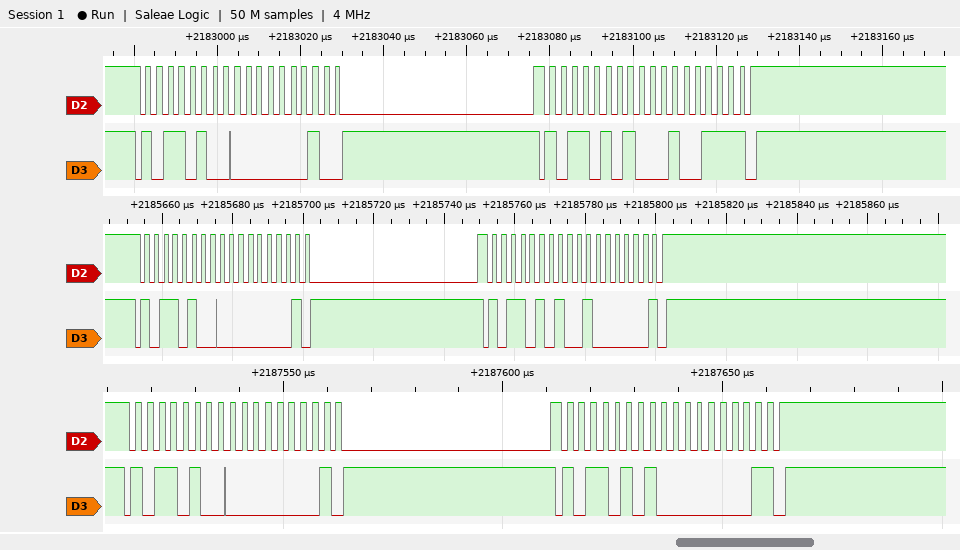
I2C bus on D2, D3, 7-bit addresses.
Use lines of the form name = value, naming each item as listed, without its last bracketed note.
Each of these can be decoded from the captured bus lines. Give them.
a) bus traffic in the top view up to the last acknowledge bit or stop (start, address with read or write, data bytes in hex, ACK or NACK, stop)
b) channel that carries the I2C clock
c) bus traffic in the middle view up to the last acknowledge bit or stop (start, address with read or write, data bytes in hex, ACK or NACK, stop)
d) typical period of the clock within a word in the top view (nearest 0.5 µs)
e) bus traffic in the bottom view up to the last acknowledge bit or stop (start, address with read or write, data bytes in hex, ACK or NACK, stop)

bus traffic in the top view up to the last acknowledge bit or stop = start, address 5A write ACK, 02 ACK, repeated start, address 5A read ACK, 27 NACK, stop
channel that carries the I2C clock = D2
bus traffic in the middle view up to the last acknowledge bit or stop = start, address 5A write ACK, 01 ACK, repeated start, address 5A read ACK, 40 NACK, stop
typical period of the clock within a word in the top view = 2.5 µs
bus traffic in the bottom view up to the last acknowledge bit or stop = start, address 5A write ACK, 01 ACK, repeated start, address 5A read ACK, 01 NACK, stop
